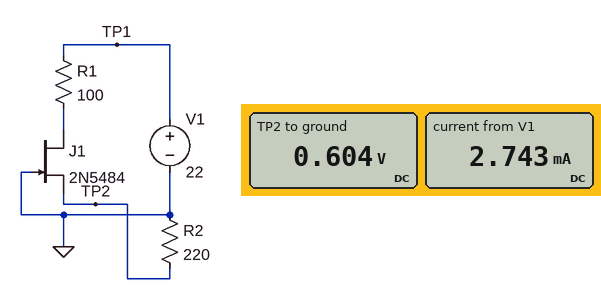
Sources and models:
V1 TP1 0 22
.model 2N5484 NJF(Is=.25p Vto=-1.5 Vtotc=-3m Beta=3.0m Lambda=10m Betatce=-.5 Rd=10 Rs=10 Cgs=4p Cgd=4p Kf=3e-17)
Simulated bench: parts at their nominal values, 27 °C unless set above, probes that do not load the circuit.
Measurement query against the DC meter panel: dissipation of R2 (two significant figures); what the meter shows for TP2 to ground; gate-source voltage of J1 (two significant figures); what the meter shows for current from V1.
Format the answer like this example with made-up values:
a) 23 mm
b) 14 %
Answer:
a) 1.7 mW
b) 0.604 V
c) -600 mV
d) 2.743 mA
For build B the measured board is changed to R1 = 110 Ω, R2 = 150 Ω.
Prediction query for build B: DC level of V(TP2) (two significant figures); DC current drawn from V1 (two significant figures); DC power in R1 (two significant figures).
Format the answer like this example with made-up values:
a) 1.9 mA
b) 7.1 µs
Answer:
a) 500 mV
b) 3.4 mA
c) 1.2 mW
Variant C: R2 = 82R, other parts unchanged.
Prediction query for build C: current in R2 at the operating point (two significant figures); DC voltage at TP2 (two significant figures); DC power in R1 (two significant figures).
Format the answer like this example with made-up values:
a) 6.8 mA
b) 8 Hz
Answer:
a) 4.4 mA
b) 360 mV
c) 1.9 mW
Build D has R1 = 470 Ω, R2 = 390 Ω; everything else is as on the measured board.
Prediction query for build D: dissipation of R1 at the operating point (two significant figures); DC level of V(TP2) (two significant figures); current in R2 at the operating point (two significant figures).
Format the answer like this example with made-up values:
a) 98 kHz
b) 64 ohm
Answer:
a) 1.7 mW
b) 750 mV
c) 1.9 mA
